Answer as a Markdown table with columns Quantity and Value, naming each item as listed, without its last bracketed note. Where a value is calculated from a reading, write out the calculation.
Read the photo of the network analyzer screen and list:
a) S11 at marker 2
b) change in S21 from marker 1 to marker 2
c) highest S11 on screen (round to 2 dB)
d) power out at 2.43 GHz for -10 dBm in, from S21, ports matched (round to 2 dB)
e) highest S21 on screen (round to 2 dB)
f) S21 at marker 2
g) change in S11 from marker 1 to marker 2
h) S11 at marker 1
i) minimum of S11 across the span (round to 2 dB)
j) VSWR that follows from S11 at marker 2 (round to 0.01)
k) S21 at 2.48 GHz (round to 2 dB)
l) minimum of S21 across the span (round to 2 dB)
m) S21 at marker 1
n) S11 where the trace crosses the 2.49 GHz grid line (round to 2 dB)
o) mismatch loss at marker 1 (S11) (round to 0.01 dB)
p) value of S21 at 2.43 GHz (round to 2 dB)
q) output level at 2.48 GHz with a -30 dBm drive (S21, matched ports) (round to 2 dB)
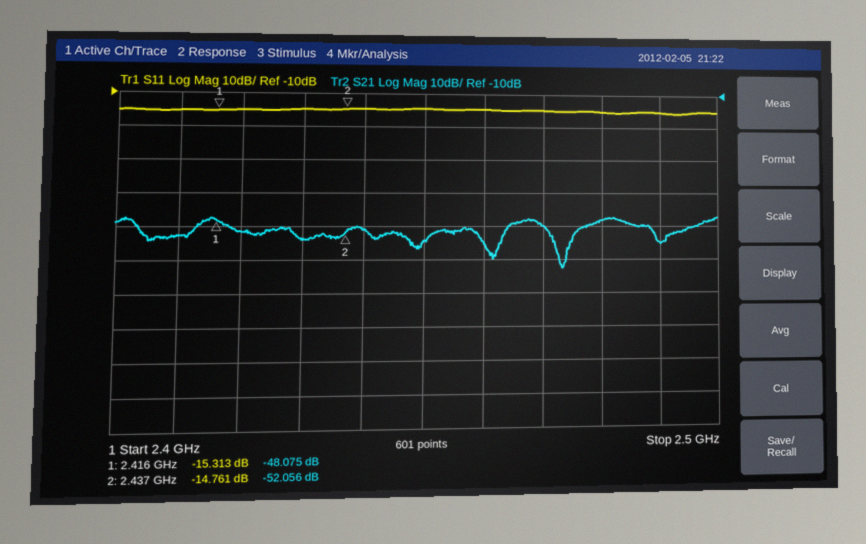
| Quantity | Value |
|---|---|
| S11 at marker 2 | -14.761 dB |
| change in S21 from marker 1 to marker 2 | -52.056 − (-48.075) = -3.981 dB |
| highest S11 on screen | -14 dB |
| power out at 2.43 GHz for -10 dBm in, from S21, ports matched | -10 dBm + (-54 dB) = -64 dBm |
| highest S21 on screen | -48 dB |
| S21 at marker 2 | -52.056 dB |
| change in S11 from marker 1 to marker 2 | -14.761 − (-15.313) = 0.552 dB |
| S11 at marker 1 | -15.313 dB |
| minimum of S11 across the span | -16 dB |
| VSWR that follows from S11 at marker 2 | (1 + 0.1828)/(1 − 0.1828) ≈ 1.45 |
| S21 at 2.48 GHz | -48 dB |
| minimum of S21 across the span | -62 dB |
| S21 at marker 1 | -48.075 dB |
| S11 where the trace crosses the 2.49 GHz grid line | -16 dB |
| mismatch loss at marker 1 (S11) | −10 log10(1 − 10^(-15.313/10)) ≈ 0.13 dB |
| value of S21 at 2.43 GHz | -54 dB |
| output level at 2.48 GHz with a -30 dBm drive (S21, matched ports) | -30 dBm + (-48 dB) = -78 dBm |
